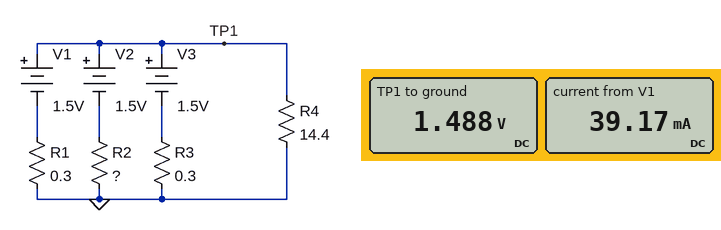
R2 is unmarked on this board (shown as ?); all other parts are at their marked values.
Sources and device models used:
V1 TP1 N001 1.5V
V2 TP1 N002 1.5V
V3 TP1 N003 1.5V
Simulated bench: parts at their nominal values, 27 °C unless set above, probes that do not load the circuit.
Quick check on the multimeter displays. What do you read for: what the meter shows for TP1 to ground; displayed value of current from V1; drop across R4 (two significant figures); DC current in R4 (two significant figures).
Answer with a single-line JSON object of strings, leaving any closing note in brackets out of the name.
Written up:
{"what the meter shows for TP1 to ground": "1.488 V", "displayed value of current from V1": "39.17 mA", "drop across R4": "1.5 V", "DC current in R4": "100 mA"}
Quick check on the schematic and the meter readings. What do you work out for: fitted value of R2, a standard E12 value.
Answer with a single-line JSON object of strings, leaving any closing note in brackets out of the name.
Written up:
{"fitted value of R2, a standard E12 value": "0.47 Ω"}
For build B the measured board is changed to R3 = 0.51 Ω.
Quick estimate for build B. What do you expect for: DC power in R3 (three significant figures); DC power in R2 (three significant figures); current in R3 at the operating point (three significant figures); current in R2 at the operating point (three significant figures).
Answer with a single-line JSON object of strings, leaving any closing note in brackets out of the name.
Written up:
{"DC power in R3": "379 µW", "DC power in R2": "411 µW", "current in R3 at the operating point": "27.3 mA", "current in R2 at the operating point": "29.6 mA"}
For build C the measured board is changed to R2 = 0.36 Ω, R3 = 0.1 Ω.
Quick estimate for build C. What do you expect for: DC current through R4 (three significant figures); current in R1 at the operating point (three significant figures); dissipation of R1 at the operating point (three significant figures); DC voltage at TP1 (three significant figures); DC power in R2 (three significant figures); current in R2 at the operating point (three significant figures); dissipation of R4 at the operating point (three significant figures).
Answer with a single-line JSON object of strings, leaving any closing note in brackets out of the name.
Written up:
{"DC current through R4": "104 mA", "current in R1 at the operating point": "21.5 mA", "dissipation of R1 at the operating point": "138 µW", "DC voltage at TP1": "1.49 V", "DC power in R2": "115 µW", "current in R2 at the operating point": "17.9 mA", "dissipation of R4 at the operating point": "155 mW"}
